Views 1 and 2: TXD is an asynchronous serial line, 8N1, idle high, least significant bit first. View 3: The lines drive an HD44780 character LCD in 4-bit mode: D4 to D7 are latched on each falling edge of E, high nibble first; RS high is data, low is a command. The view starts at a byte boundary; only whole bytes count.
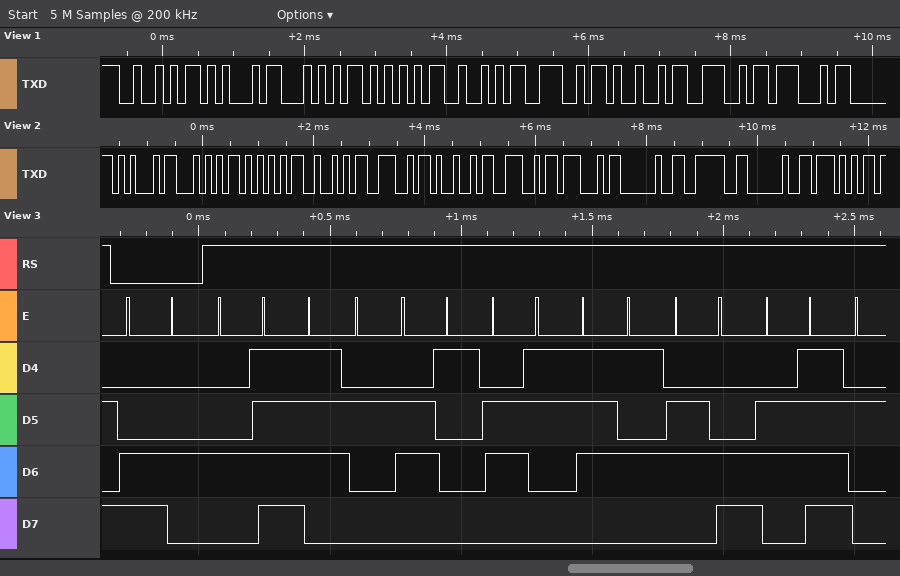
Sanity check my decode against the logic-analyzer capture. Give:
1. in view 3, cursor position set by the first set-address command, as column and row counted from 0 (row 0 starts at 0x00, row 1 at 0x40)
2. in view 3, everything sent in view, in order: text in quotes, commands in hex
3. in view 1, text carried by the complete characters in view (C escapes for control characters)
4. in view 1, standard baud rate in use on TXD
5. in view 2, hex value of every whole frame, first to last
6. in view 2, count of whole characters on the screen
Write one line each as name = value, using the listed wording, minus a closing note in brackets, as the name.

in view 3, cursor position set by the first set-address command, as column and row counted from 0 = column 4, row 1
in view 3, everything sent in view, in order: text in quotes, commands in hex = 0xC4 "Oraculo"
in view 1, text carried by the complete characters in view = "RETURNING"
in view 1, standard baud rate in use on TXD = 9600 baud
in view 2, hex value of every whole frame, first to last = 45 54 55 52 4E 49 4E 47 20 3E 20 57
in view 2, count of whole characters on the screen = 12
